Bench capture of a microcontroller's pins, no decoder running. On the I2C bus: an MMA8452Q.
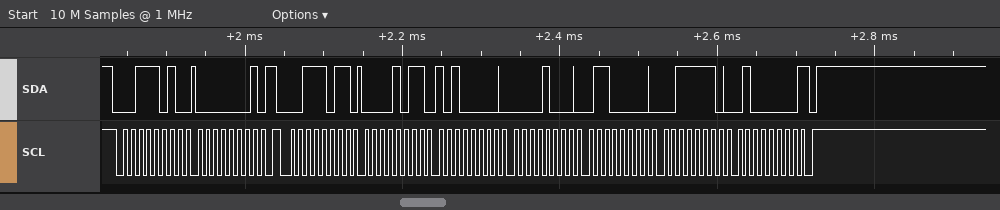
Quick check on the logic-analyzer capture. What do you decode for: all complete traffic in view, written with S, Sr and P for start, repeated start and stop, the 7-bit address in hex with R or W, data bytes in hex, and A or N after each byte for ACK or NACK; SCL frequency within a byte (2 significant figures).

S 1DW A 01 A Sr 1DR A 0B A A0 A 08 A 60 A 3E A 40 N P
100 kHz
